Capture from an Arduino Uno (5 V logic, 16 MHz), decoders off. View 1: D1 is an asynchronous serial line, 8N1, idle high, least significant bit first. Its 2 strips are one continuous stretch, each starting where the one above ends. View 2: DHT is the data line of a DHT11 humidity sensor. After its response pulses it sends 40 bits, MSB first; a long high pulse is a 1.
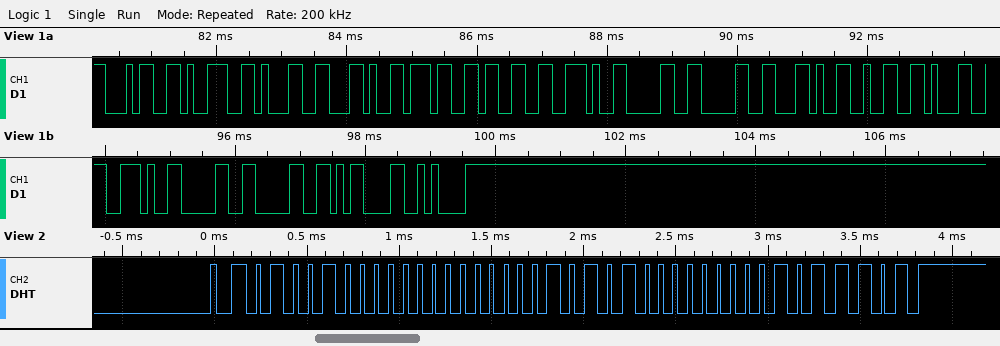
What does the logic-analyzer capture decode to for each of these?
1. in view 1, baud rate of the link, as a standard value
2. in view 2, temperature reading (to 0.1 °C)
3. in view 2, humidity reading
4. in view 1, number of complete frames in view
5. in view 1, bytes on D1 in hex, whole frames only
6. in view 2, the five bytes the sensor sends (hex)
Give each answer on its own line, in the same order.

9600 baud
21.0 °C
72 %
17
34 39 31 2C 37 33 2E 30 30 2C 32 31 2E 30 30 0D 0A
48 00 15 00 5D
